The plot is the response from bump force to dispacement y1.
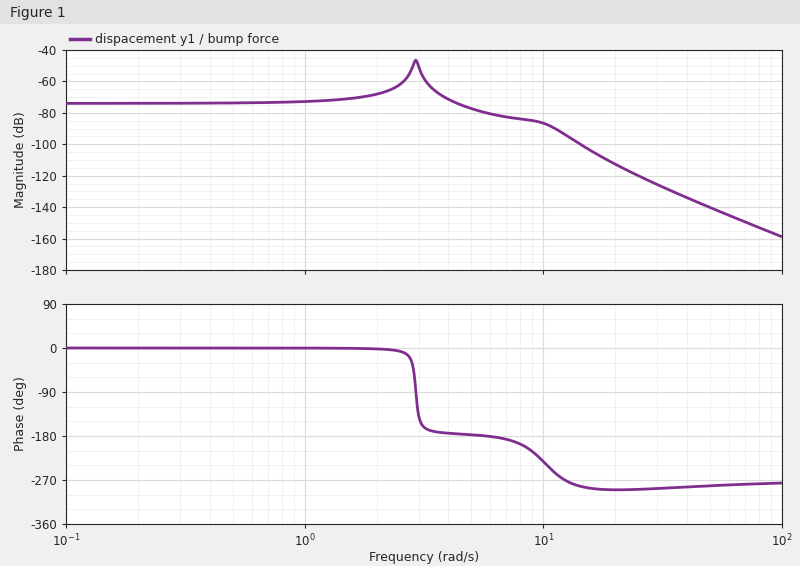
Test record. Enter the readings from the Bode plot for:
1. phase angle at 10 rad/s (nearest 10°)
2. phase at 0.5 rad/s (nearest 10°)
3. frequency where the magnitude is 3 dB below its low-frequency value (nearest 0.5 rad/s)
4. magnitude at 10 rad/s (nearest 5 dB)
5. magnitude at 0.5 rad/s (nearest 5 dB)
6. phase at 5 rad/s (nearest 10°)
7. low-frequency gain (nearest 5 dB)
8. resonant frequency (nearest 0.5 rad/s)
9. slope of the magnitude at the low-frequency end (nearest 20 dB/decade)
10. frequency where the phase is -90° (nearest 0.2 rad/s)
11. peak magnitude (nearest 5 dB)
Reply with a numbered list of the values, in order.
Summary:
1. -230°
2. 0°
3. 5.0 rad/s
4. -85 dB
5. -75 dB
6. -180°
7. -75 dB
8. 3.0 rad/s
9. 0 dB/decade
10. 3.0 rad/s
11. -45 dB
